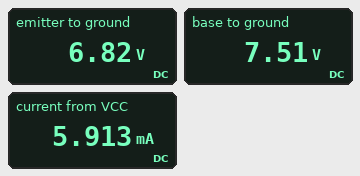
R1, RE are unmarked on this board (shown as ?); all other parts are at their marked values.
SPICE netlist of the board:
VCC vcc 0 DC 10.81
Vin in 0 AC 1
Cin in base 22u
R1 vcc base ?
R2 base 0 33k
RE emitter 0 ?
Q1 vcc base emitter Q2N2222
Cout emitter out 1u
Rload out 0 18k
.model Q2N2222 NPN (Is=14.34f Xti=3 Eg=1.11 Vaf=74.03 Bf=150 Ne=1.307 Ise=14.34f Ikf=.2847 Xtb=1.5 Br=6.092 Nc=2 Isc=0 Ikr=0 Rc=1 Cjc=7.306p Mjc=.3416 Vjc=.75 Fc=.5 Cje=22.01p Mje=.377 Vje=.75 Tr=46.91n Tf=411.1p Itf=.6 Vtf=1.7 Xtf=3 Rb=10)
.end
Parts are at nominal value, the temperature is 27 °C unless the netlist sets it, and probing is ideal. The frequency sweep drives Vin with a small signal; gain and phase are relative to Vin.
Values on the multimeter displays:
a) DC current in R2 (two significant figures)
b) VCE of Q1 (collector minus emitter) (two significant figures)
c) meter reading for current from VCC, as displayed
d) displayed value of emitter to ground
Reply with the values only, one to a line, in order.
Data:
230 µA
4.0 V
5.913 mA
6.82 V
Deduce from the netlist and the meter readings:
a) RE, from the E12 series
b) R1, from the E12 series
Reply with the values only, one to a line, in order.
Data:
1.2 kΩ
12 kΩ
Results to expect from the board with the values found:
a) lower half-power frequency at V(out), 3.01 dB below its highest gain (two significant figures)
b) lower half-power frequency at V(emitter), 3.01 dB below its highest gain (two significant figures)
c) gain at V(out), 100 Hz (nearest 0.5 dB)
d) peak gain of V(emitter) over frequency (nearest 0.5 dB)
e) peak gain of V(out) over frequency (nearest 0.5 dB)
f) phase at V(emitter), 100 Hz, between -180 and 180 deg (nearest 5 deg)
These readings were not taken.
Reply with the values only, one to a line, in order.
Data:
8.9 Hz
870 mHz
0 dB
0 dB
0 dB
0 deg
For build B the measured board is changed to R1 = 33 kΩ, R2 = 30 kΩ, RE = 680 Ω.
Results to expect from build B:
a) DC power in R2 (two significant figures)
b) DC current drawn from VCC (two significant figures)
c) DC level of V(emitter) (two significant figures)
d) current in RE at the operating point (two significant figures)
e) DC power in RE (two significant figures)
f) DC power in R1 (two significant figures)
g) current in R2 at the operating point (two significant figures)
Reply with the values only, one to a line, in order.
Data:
660 µW
5.7 mA
3.8 V
5.5 mA
21 mW
1.2 mW
150 µA
